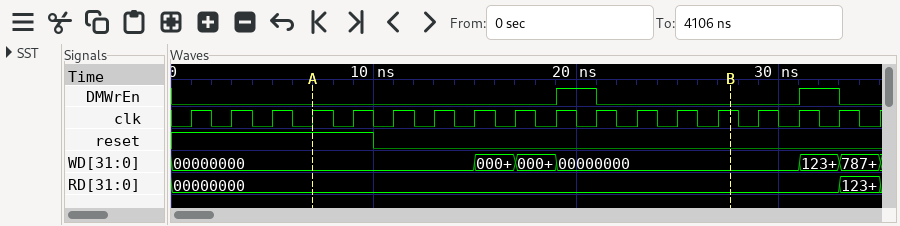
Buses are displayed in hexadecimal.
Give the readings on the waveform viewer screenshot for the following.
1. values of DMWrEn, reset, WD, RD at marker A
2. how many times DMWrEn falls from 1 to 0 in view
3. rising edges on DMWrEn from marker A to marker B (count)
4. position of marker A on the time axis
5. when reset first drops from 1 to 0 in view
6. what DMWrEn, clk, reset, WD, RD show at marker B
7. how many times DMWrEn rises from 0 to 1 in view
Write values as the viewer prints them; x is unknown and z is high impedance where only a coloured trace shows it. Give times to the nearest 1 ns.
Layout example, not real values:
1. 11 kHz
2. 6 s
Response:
1. DMWrEn=0, reset=1, WD=00000000, RD=00000000
2. 2
3. 1
4. 7 ns
5. 10 ns
6. DMWrEn=0, clk=1, reset=0, WD=00000000, RD=00000000
7. 2
